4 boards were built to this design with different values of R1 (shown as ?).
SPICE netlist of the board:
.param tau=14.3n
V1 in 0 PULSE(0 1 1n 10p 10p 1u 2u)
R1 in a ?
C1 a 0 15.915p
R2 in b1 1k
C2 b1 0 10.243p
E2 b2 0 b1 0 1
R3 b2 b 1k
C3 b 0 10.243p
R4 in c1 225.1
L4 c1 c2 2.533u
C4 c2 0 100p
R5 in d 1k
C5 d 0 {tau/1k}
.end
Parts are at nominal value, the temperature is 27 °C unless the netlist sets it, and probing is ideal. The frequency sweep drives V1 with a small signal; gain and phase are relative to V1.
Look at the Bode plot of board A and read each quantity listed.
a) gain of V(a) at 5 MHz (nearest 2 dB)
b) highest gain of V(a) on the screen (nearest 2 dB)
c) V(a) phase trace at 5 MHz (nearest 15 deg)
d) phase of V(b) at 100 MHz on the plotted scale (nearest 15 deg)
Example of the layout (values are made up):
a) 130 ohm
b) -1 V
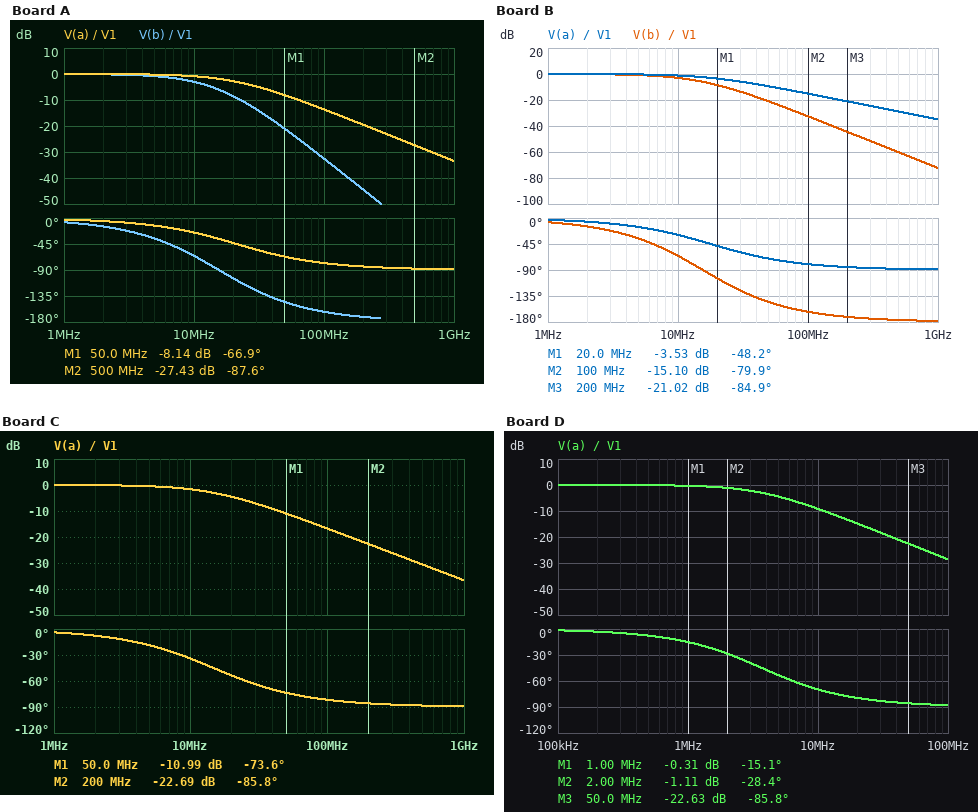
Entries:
a) 0 dB
b) 0 dB
c) -15 deg
d) -165 deg
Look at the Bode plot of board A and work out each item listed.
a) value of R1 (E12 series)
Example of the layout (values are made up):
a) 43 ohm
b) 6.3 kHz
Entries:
a) 470 Ω
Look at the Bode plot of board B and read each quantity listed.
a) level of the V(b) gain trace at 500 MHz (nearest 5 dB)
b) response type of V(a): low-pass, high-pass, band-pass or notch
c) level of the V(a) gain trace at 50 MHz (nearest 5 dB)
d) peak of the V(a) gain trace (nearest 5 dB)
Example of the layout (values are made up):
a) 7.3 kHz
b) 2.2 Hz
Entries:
a) -60 dB
b) low-pass
c) -10 dB
d) 0 dB
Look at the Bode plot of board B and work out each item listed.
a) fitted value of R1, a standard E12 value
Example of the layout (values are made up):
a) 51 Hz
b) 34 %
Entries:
a) 560 Ω
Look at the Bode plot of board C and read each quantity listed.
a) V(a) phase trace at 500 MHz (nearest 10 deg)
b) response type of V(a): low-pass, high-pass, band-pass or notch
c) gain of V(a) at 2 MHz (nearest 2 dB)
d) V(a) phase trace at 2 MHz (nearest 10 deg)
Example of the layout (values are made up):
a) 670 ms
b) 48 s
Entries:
a) -90 deg
b) low-pass
c) 0 dB
d) -10 deg
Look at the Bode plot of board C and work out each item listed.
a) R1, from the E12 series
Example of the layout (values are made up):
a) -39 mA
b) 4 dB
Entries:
a) 680 Ω
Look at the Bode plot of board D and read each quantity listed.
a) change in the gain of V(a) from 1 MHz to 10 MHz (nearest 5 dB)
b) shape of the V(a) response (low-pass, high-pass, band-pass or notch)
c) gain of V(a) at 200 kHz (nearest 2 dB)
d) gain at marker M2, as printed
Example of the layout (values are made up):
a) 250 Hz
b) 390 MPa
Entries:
a) -10 dB
b) low-pass
c) 0 dB
d) -1.11 dB
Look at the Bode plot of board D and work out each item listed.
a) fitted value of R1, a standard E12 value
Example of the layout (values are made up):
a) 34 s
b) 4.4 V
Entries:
a) 2.7 kΩ
